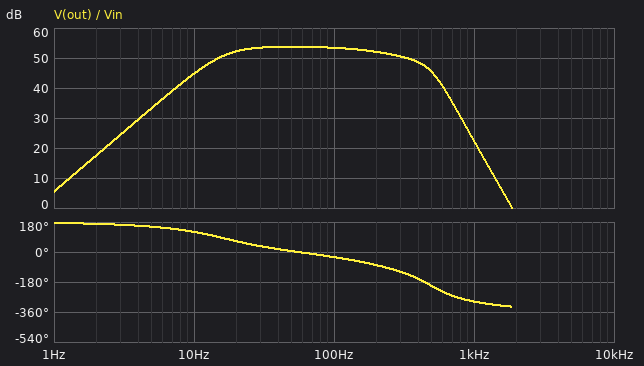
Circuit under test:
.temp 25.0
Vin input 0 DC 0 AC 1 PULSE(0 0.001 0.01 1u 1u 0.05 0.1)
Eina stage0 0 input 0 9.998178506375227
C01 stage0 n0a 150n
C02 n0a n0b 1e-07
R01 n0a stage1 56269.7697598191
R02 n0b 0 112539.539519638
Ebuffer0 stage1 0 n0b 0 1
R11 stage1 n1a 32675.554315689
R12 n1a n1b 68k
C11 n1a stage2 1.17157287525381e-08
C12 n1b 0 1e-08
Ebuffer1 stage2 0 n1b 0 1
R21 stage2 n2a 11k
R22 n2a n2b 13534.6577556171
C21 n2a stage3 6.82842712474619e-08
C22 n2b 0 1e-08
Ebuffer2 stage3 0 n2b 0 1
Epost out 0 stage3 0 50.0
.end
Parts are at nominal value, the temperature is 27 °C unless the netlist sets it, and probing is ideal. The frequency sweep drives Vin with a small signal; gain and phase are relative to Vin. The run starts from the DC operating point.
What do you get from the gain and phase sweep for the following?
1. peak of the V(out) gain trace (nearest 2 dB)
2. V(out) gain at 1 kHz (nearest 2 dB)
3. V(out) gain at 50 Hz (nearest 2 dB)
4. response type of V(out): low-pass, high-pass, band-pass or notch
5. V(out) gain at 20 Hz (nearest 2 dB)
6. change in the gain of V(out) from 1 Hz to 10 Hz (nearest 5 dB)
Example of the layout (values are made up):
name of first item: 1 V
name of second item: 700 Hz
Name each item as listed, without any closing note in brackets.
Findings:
peak of the V(out) gain trace: 54 dB
V(out) gain at 1 kHz: 22 dB
V(out) gain at 50 Hz: 54 dB
response type of V(out): low-pass, high-pass, band-pass or notch: band-pass
V(out) gain at 20 Hz: 52 dB
change in the gain of V(out) from 1 Hz to 10 Hz: 40 dB
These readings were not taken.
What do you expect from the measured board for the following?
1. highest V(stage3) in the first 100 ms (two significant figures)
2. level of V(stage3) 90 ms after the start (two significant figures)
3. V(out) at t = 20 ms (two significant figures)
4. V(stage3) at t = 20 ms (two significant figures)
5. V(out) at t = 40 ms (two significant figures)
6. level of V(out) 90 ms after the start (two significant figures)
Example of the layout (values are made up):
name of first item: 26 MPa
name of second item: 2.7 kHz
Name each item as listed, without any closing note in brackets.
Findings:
highest V(stage3) in the first 100 ms: 8.2 mV
level of V(stage3) 90 ms after the start: 1.7 mV
V(out) at t = 20 ms: 55 mV
V(stage3) at t = 20 ms: 1.1 mV
V(out) at t = 40 ms: -82 mV
level of V(out) 90 ms after the start: 84 mV
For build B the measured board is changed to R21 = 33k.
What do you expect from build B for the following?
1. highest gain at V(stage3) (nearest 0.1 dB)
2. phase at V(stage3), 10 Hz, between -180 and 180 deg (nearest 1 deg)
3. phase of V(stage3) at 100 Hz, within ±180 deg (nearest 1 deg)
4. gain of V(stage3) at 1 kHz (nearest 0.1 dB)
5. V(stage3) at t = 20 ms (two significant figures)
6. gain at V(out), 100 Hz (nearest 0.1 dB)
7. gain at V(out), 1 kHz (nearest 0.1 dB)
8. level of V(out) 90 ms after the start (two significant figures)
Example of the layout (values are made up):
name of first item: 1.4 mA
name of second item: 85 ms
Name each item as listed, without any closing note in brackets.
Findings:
highest gain at V(stage3): 19.9 dB
phase at V(stage3), 10 Hz, between -180 and 180 deg: 120 deg
phase of V(stage3) at 100 Hz, within ±180 deg: -40 deg
gain of V(stage3) at 1 kHz: -22.2 dB
V(stage3) at t = 20 ms: 1.2 mV
gain at V(out), 100 Hz: 53.8 dB
gain at V(out), 1 kHz: 11.8 dB
level of V(out) 90 ms after the start: 85 mV
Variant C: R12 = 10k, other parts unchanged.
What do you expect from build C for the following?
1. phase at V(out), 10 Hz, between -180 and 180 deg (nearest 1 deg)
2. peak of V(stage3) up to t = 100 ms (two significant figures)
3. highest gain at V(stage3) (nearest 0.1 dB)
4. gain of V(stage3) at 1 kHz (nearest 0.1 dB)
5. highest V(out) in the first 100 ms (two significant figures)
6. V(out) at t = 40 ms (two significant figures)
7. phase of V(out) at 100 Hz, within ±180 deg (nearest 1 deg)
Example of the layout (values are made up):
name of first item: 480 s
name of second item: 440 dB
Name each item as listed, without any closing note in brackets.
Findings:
phase at V(out), 10 Hz, between -180 and 180 deg: 123 deg
peak of V(stage3) up to t = 100 ms: 10 mV
highest gain at V(stage3): 20.7 dB
gain of V(stage3) at 1 kHz: 0.7 dB
highest V(out) in the first 100 ms: 520 mV
V(out) at t = 40 ms: -80 mV
phase of V(out) at 100 Hz, within ±180 deg: -11 deg
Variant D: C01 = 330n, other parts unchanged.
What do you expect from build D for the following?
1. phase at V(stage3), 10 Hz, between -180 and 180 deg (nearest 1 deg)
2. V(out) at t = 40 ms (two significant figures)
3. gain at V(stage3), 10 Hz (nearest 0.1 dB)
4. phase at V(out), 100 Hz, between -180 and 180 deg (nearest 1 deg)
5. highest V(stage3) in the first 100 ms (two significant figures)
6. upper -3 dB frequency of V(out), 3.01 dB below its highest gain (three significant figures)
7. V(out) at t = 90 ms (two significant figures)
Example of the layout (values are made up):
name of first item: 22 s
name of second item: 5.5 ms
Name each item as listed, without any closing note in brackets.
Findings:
phase at V(stage3), 10 Hz, between -180 and 180 deg: 92 deg
V(out) at t = 40 ms: -84 mV
gain at V(stage3), 10 Hz: 14.6 dB
phase at V(out), 100 Hz, between -180 and 180 deg: -34 deg
highest V(stage3) in the first 100 ms: 8.5 mV
upper -3 dB frequency of V(out), 3.01 dB below its highest gain: 289 Hz
V(out) at t = 90 ms: 78 mV
